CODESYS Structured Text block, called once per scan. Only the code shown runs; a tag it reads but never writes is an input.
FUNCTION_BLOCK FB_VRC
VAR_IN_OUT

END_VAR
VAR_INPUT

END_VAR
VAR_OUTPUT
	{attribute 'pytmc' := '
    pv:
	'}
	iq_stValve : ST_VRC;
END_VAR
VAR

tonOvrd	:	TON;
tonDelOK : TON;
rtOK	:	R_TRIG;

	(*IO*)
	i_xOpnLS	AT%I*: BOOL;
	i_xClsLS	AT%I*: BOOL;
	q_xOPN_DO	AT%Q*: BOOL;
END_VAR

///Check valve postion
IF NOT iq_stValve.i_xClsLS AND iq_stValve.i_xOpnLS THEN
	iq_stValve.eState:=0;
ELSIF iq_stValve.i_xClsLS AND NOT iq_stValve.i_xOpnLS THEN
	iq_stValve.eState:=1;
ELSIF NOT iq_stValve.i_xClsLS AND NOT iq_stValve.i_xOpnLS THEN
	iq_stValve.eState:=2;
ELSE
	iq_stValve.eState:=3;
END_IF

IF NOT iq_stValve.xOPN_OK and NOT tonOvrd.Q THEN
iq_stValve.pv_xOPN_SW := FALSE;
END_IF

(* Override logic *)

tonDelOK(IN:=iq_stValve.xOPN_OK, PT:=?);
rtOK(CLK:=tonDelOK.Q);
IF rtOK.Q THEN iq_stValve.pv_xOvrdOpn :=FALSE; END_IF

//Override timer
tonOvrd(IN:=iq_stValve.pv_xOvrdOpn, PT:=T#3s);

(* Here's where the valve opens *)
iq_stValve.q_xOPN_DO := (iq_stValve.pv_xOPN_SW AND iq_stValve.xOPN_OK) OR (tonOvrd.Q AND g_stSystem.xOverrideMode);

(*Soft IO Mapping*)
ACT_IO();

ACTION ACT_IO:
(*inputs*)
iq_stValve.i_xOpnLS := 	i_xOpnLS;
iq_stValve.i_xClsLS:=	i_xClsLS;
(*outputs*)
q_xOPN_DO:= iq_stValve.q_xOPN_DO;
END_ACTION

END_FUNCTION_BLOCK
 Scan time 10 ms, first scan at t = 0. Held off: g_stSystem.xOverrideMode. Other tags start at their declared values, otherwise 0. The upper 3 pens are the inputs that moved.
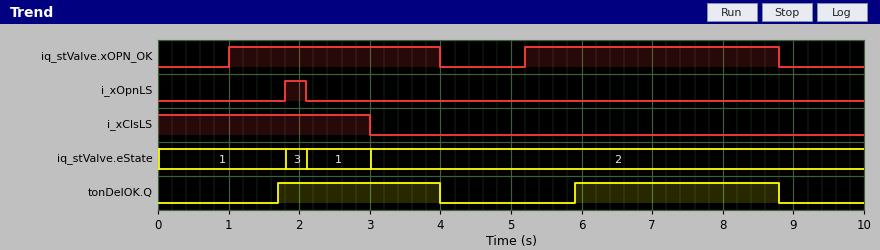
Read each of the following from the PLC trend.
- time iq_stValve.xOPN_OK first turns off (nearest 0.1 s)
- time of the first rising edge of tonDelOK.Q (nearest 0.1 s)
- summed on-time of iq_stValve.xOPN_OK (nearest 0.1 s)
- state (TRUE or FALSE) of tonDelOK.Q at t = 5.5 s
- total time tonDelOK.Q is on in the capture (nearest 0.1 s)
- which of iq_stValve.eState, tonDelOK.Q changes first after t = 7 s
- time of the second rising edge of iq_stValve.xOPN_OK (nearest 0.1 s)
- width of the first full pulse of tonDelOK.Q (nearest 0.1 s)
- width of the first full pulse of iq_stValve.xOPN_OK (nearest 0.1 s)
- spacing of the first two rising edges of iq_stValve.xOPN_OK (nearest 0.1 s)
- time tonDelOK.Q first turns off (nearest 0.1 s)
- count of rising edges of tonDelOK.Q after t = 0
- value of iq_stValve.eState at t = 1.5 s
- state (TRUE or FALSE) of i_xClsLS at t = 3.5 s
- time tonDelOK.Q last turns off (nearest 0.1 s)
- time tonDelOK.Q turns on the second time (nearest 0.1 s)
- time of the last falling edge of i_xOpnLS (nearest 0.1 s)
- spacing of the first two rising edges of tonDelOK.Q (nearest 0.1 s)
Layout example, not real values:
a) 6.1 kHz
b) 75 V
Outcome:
a) 4.0 s
b) 1.7 s
c) 6.6 s
d) FALSE
e) 5.2 s
f) tonDelOK.Q
g) 5.2 s
h) 2.3 s
i) 3.0 s
j) 4.2 s
k) 4.0 s
l) 2
m) 1
n) FALSE
o) 8.8 s
p) 5.9 s
q) 2.1 s
r) 4.2 s
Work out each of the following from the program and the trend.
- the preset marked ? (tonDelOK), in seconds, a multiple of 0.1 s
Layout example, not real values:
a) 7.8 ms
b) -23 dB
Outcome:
a) 0.7 s
